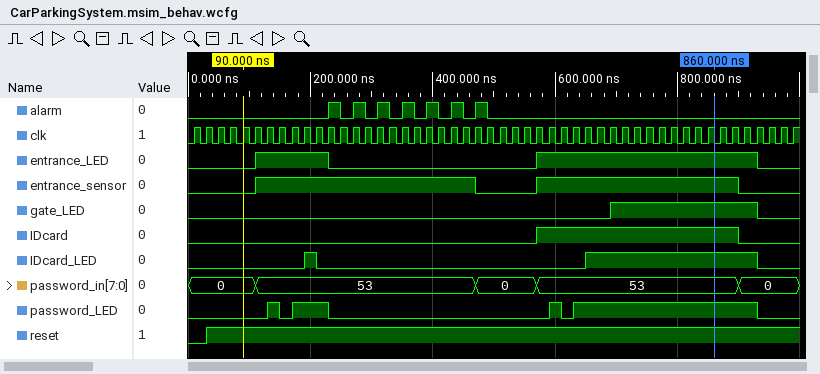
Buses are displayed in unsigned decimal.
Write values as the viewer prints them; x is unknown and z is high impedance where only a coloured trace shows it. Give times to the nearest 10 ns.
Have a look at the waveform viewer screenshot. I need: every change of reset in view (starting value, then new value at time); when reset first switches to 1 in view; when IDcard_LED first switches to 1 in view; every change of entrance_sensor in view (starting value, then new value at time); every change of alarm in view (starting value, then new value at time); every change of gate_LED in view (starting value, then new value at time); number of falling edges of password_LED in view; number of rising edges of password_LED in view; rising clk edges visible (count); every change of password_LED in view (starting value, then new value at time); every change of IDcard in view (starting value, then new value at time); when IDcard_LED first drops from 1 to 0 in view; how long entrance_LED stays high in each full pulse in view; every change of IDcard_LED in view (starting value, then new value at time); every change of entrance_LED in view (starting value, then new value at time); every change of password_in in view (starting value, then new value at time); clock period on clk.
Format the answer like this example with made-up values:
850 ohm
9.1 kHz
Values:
0, 1 at 30 ns
30 ns
190 ns
0, 1 at 110 ns, 0 at 470 ns, 1 at 570 ns, 0 at 900 ns
0, 1 at 230 ns, 0 at 250 ns, 1 at 270 ns, 0 at 290 ns, 1 at 310 ns, 0 at 330 ns, 1 at 350 ns, 0 at 370 ns, 1 at 390 ns, 0 at 410 ns, 1 at 430 ns, 0 at 450 ns, 1 at 470 ns, 0 at 490 ns
0, 1 at 690 ns, 0 at 930 ns
4
4
50
0, 1 at 130 ns, 0 at 150 ns, 1 at 170 ns, 0 at 230 ns, 1 at 590 ns, 0 at 610 ns, 1 at 630 ns, 0 at 930 ns
0, 1 at 570 ns, 0 at 900 ns
210 ns
120 ns, 360 ns
0, 1 at 190 ns, 0 at 210 ns, 1 at 650 ns, 0 at 930 ns
0, 1 at 110 ns, 0 at 230 ns, 1 at 570 ns, 0 at 930 ns
0, 53 at 110 ns, 0 at 470 ns, 53 at 570 ns, 0 at 900 ns
20 ns
